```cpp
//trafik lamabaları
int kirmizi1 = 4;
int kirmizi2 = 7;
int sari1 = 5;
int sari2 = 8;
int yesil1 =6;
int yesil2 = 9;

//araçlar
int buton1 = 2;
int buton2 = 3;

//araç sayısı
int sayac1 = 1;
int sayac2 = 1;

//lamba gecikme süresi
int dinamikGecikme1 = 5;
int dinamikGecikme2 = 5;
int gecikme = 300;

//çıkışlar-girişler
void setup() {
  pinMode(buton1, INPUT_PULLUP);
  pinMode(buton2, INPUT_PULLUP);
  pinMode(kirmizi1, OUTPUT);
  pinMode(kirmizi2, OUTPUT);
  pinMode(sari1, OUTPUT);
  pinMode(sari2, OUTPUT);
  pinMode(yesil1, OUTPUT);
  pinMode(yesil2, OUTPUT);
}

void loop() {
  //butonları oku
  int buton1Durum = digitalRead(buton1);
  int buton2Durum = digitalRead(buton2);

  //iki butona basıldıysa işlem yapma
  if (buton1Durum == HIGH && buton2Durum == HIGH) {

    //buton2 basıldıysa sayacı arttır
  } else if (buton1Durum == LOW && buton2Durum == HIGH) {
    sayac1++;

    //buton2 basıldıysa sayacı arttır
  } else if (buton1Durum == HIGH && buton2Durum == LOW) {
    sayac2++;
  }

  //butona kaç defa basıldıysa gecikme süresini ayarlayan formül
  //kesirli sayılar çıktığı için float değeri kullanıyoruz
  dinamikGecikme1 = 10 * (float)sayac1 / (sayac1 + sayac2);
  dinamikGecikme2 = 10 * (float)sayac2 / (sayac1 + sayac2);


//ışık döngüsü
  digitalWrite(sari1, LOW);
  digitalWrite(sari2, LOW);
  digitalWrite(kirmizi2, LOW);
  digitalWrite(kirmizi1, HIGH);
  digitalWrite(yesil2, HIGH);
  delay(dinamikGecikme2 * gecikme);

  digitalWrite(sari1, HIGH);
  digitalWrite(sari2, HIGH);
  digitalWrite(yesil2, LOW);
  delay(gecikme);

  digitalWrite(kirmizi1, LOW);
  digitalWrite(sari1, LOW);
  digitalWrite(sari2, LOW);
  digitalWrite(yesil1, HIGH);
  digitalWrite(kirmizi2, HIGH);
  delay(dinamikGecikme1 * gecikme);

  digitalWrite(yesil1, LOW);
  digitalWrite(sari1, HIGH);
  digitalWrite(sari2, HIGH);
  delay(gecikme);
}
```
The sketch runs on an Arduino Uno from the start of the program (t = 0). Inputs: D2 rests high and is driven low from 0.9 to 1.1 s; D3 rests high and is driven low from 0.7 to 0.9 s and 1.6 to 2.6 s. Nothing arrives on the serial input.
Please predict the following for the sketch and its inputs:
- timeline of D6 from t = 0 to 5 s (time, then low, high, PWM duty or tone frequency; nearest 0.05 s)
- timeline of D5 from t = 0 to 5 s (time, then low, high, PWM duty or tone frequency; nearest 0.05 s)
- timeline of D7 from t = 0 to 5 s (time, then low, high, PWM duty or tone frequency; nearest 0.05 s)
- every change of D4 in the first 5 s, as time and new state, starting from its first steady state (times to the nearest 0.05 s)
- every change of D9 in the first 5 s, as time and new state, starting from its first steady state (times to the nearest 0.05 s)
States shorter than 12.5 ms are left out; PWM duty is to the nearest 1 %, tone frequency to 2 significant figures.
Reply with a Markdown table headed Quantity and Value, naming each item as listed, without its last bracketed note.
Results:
| Quantity | Value |
|---|---|
| timeline of D6 from t = 0 to 5 s | 0 s low; 1.8 s high; 3.3 s low |
| timeline of D5 from t = 0 to 5 s | 0 s low; 1.5 s high; 1.8 s low; 3.3 s high; 3.6 s low |
| timeline of D7 from t = 0 to 5 s | 0 s low; 1.8 s high; 3.6 s low |
| every change of D4 in the first 5 s, as time and new state, starting from its first steady state | 0 s high; 1.8 s low; 3.6 s high |
| every change of D9 in the first 5 s, as time and new state, starting from its first steady state | 0 s high; 1.5 s low; 3.6 s high |
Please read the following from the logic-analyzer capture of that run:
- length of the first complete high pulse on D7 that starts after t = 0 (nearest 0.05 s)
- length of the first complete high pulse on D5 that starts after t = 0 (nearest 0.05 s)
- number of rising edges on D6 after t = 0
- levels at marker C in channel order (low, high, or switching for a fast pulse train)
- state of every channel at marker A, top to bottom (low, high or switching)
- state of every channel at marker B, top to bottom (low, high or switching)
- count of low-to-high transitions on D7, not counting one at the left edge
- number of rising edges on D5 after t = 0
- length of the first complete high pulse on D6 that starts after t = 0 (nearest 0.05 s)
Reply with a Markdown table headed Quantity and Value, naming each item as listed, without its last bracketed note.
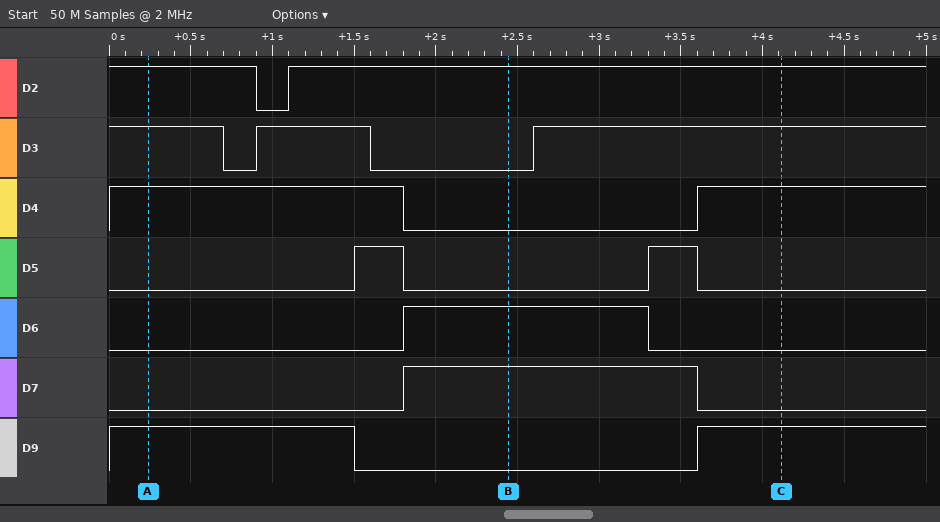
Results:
| Quantity | Value |
|---|---|
| length of the first complete high pulse on D7 that starts after t = 0 | 1.80 s |
| length of the first complete high pulse on D5 that starts after t = 0 | 0.30 s |
| number of rising edges on D6 after t = 0 | 1 |
| levels at marker C in channel order | D2 high, D3 high, D4 high, D5 low, D6 low, D7 low, D9 high |
| state of every channel at marker A, top to bottom | D2 high, D3 high, D4 high, D5 low, D6 low, D7 low, D9 high |
| state of every channel at marker B, top to bottom | D2 high, D3 low, D4 low, D5 low, D6 high, D7 high, D9 low |
| count of low-to-high transitions on D7, not counting one at the left edge | 1 |
| number of rising edges on D5 after t = 0 | 2 |
| length of the first complete high pulse on D6 that starts after t = 0 | 1.50 s |
